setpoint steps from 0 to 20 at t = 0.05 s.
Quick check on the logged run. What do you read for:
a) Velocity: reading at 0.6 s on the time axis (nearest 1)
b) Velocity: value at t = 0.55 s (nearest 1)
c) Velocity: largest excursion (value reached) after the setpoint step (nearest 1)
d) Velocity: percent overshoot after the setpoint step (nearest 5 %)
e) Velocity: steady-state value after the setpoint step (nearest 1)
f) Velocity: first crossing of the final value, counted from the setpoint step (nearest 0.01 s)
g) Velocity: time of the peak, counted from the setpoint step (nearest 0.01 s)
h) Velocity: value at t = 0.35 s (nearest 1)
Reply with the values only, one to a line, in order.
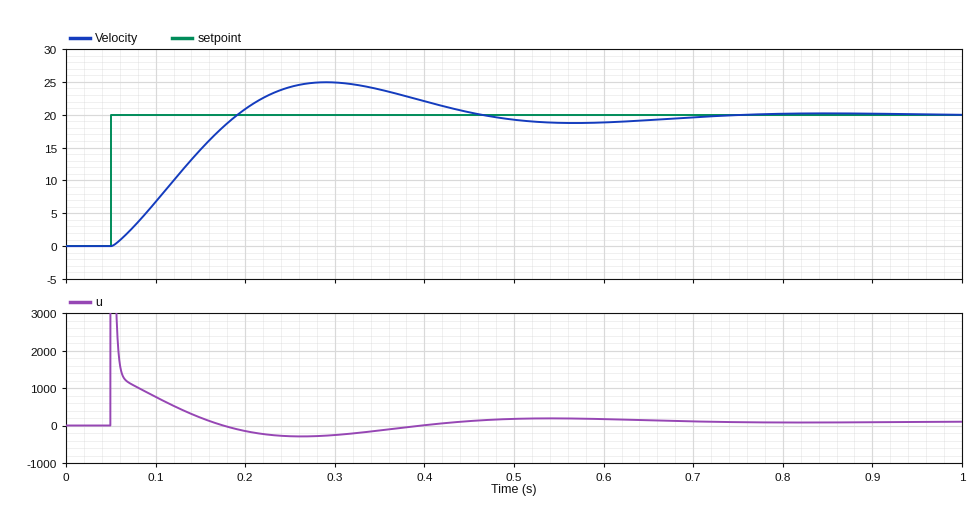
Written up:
19
19
25
25 %
20
0.14 s
0.24 s
24
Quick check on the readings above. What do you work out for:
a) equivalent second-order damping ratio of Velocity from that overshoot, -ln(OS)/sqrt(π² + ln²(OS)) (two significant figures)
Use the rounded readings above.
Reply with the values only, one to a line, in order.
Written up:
0.40
